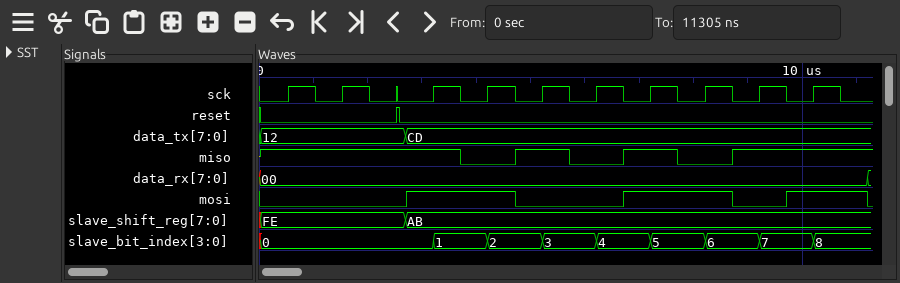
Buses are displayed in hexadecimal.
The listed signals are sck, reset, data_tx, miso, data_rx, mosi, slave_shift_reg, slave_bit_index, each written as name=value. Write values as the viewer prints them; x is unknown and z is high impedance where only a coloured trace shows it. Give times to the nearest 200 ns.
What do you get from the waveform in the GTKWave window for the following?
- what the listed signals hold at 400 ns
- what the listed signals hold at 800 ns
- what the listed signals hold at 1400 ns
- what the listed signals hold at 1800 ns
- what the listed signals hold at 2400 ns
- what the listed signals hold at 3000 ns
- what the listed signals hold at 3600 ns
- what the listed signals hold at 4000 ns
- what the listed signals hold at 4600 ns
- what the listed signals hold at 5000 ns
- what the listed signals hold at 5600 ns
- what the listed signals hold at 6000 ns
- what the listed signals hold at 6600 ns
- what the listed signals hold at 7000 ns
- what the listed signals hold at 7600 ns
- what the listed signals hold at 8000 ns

sck=0, reset=0, data_tx=12, miso=1, data_rx=00, mosi=0, slave_shift_reg=FE, slave_bit_index=0
sck=1, reset=0, data_tx=12, miso=1, data_rx=00, mosi=0, slave_shift_reg=FE, slave_bit_index=0
sck=0, reset=0, data_tx=12, miso=1, data_rx=00, mosi=0, slave_shift_reg=FE, slave_bit_index=0
sck=1, reset=0, data_tx=12, miso=1, data_rx=00, mosi=0, slave_shift_reg=FE, slave_bit_index=0
sck=0, reset=0, data_tx=12, miso=1, data_rx=00, mosi=0, slave_shift_reg=FE, slave_bit_index=0
sck=0, reset=0, data_tx=CD, miso=1, data_rx=00, mosi=1, slave_shift_reg=AB, slave_bit_index=0
sck=1, reset=0, data_tx=CD, miso=1, data_rx=00, mosi=1, slave_shift_reg=AB, slave_bit_index=1
sck=0, reset=0, data_tx=CD, miso=0, data_rx=00, mosi=1, slave_shift_reg=AB, slave_bit_index=1
sck=1, reset=0, data_tx=CD, miso=0, data_rx=00, mosi=1, slave_shift_reg=AB, slave_bit_index=2
sck=0, reset=0, data_tx=CD, miso=1, data_rx=00, mosi=0, slave_shift_reg=AB, slave_bit_index=2
sck=1, reset=0, data_tx=CD, miso=1, data_rx=00, mosi=0, slave_shift_reg=AB, slave_bit_index=3
sck=0, reset=0, data_tx=CD, miso=0, data_rx=00, mosi=0, slave_shift_reg=AB, slave_bit_index=3
sck=1, reset=0, data_tx=CD, miso=0, data_rx=00, mosi=0, slave_shift_reg=AB, slave_bit_index=4
sck=0, reset=0, data_tx=CD, miso=1, data_rx=00, mosi=1, slave_shift_reg=AB, slave_bit_index=4
sck=1, reset=0, data_tx=CD, miso=1, data_rx=00, mosi=1, slave_shift_reg=AB, slave_bit_index=5
sck=0, reset=0, data_tx=CD, miso=0, data_rx=00, mosi=1, slave_shift_reg=AB, slave_bit_index=5
